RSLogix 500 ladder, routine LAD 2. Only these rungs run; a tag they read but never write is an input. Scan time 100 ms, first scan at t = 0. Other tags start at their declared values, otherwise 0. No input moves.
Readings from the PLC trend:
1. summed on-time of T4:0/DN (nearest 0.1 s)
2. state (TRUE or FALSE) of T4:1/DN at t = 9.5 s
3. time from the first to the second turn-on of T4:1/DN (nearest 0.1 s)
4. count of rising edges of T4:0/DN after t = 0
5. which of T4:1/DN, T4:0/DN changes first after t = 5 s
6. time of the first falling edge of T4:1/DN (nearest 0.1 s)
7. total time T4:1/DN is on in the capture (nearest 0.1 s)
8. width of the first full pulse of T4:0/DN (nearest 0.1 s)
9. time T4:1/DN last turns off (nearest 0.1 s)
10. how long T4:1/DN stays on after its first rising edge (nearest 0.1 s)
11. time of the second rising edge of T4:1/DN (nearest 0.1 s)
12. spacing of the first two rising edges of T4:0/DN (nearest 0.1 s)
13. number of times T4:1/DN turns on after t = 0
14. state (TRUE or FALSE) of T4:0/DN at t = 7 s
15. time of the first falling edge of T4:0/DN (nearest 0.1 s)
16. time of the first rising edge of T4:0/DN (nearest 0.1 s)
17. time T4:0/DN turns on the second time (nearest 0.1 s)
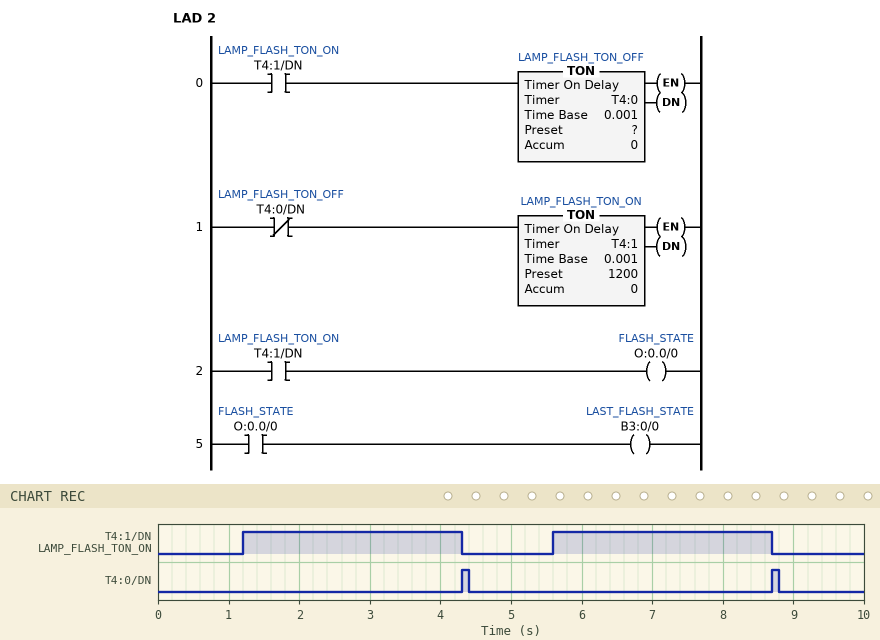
0.2 s
FALSE
4.4 s
2
T4:1/DN
4.3 s
6.2 s
0.1 s
8.7 s
3.1 s
5.6 s
4.4 s
2
FALSE
4.4 s
4.3 s
8.7 s
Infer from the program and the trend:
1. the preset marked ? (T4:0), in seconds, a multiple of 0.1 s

3.0 s
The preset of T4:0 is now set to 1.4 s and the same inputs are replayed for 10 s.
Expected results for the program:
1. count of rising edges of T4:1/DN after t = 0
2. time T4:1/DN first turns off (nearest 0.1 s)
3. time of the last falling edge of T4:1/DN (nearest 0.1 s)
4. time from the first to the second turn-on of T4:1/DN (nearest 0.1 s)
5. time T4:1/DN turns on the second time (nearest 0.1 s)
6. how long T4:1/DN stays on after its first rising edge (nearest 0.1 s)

4
2.7 s
8.3 s
2.8 s
4.0 s
1.5 s
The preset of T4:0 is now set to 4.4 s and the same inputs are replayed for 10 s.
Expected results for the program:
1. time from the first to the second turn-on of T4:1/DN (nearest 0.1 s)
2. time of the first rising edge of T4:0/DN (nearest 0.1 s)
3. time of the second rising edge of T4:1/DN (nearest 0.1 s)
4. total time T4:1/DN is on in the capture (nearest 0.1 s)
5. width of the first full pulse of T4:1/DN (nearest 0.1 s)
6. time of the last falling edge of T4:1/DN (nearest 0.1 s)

5.8 s
5.7 s
7.0 s
7.5 s
4.5 s
5.7 s
